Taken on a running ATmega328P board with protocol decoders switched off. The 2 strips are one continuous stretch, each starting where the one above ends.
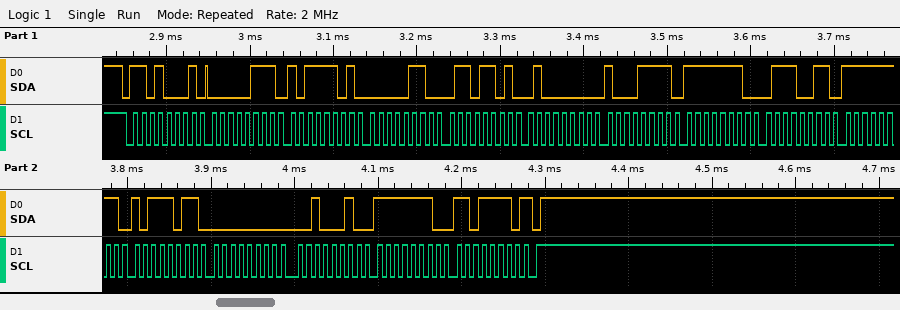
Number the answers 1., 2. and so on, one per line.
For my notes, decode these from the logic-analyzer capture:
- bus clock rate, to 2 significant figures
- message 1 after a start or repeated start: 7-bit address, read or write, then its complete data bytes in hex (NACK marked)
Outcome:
1. 100 kHz
2. 0x68 read: 07 BD 06 6D 40 8F FE 73 FF BB 00 22 FE DE NACK
